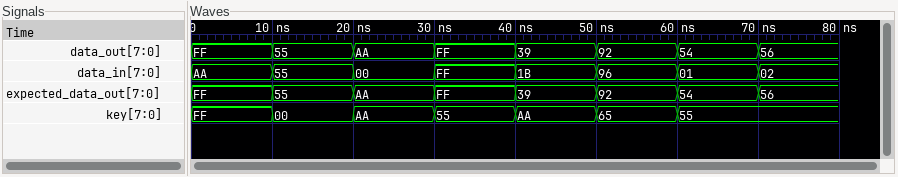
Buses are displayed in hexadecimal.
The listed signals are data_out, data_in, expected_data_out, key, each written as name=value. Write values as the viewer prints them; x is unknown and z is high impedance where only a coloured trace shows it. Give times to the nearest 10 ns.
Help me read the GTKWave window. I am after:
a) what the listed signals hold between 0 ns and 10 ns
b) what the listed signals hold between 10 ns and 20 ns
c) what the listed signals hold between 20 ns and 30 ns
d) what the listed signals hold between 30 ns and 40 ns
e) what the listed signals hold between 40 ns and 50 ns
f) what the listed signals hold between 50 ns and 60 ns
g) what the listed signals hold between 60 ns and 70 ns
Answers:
data_out=FF, data_in=AA, expected_data_out=FF, key=FF
data_out=55, data_in=55, expected_data_out=55, key=00
data_out=AA, data_in=00, expected_data_out=AA, key=AA
data_out=FF, data_in=FF, expected_data_out=FF, key=55
data_out=39, data_in=1B, expected_data_out=39, key=AA
data_out=92, data_in=96, expected_data_out=92, key=65
data_out=54, data_in=01, expected_data_out=54, key=55
